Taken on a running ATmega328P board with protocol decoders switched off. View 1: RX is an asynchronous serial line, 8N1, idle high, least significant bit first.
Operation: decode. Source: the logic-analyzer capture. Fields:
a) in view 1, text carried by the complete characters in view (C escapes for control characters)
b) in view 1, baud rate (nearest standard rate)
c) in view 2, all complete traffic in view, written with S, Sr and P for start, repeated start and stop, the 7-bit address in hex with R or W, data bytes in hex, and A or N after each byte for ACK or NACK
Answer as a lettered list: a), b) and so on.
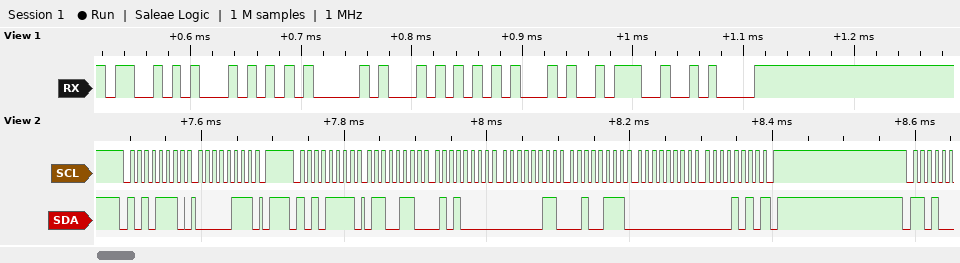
a) "STATE:\n"
b) 115200 baud
c) S 57W A 07 A P S 57R A 66 A 50 A 03 A 27 A 00 A 0A N P
